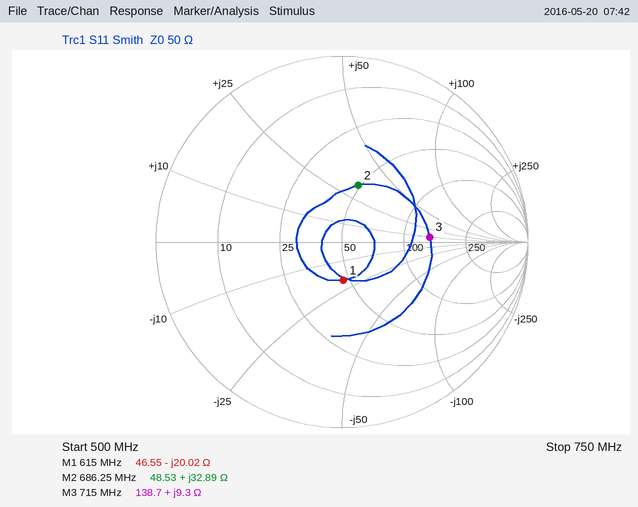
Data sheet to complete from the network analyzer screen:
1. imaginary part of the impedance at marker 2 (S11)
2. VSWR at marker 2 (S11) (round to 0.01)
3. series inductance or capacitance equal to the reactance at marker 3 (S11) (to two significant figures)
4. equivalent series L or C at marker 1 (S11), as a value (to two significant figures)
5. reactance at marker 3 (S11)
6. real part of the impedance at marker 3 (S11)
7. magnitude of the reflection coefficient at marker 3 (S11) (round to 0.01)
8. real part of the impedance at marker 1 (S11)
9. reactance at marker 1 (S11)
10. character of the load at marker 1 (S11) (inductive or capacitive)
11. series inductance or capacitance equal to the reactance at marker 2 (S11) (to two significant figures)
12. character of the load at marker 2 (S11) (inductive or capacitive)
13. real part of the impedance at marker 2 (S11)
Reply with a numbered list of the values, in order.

1. +32.89 Ω
2. 1.93
3. 2.1 nH
4. 13 pF
5. +9.3 Ω
6. 138.7 Ω
7. 0.47
8. 46.55 Ω
9. -20.02 Ω
10. capacitive
11. 7.6 nH
12. inductive
13. 48.53 Ω
